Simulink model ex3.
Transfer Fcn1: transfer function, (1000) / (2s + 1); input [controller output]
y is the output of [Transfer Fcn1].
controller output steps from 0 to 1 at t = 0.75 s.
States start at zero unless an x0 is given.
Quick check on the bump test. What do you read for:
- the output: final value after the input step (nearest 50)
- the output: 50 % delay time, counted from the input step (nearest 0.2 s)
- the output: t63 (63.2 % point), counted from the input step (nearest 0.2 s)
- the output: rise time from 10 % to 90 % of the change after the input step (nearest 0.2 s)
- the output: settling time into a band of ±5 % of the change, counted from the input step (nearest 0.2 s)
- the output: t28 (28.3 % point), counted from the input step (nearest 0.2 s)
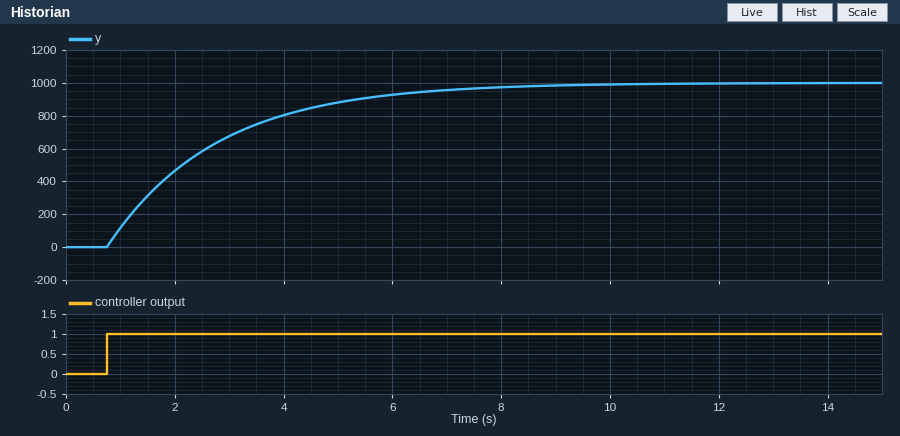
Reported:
1000
1.4 s
2.0 s
4.4 s
6.0 s
0.6 s
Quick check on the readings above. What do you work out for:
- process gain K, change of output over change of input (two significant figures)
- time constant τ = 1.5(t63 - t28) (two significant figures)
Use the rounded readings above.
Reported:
1000
2.1 s
